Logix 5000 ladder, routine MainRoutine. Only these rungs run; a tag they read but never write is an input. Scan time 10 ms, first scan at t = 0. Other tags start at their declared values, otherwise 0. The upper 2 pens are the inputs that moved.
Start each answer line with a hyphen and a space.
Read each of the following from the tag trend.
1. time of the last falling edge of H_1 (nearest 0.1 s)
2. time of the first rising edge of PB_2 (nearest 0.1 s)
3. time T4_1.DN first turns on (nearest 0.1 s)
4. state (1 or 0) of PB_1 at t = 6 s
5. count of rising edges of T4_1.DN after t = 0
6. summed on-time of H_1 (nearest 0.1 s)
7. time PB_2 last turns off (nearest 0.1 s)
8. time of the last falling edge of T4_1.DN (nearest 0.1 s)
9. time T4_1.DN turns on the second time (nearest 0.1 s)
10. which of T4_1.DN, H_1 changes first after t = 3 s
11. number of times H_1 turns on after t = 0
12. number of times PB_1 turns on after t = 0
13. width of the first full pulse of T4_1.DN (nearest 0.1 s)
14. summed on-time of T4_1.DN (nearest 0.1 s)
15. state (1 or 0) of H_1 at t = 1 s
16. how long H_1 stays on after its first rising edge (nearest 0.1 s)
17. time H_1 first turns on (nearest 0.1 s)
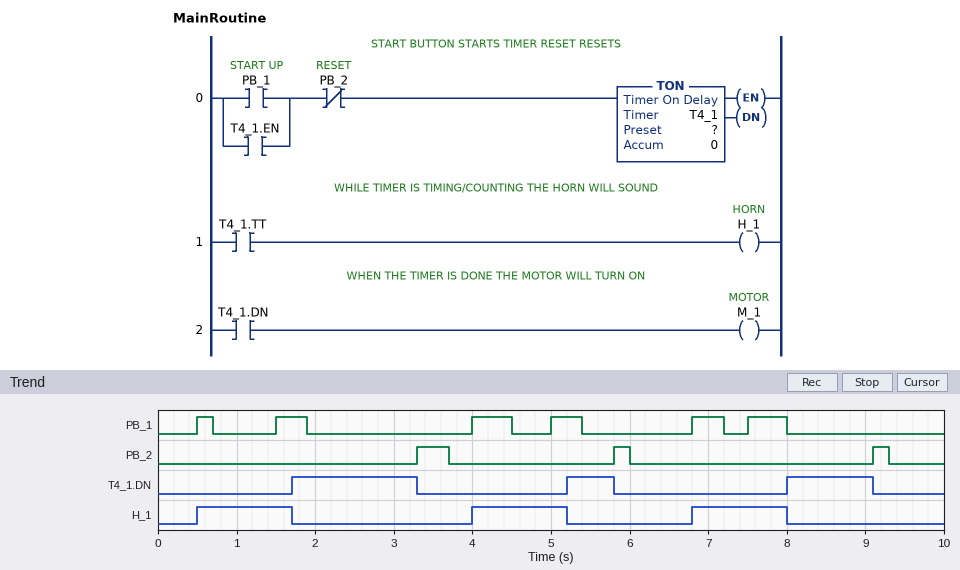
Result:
- 8.0 s
- 3.3 s
- 1.7 s
- 0
- 3
- 3.6 s
- 9.3 s
- 9.1 s
- 5.2 s
- T4_1.DN
- 3
- 6
- 1.6 s
- 3.3 s
- 1
- 1.2 s
- 0.5 s
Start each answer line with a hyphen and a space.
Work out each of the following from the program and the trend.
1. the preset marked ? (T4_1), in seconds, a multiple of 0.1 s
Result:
- 1.2 s
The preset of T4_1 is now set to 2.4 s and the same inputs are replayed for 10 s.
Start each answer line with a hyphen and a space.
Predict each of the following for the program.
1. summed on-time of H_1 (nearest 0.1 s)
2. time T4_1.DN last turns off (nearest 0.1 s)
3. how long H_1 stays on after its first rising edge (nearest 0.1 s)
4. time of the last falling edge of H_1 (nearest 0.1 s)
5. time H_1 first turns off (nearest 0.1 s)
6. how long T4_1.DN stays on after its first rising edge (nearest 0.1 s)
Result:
- 6.5 s
- 3.3 s
- 2.4 s
- 9.1 s
- 2.9 s
- 0.4 s
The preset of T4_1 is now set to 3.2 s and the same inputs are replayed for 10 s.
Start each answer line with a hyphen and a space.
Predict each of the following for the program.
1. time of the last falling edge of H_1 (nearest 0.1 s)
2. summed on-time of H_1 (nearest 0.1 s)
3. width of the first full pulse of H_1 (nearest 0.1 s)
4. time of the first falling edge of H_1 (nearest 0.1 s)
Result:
- 9.1 s
- 6.9 s
- 2.8 s
- 3.3 s
